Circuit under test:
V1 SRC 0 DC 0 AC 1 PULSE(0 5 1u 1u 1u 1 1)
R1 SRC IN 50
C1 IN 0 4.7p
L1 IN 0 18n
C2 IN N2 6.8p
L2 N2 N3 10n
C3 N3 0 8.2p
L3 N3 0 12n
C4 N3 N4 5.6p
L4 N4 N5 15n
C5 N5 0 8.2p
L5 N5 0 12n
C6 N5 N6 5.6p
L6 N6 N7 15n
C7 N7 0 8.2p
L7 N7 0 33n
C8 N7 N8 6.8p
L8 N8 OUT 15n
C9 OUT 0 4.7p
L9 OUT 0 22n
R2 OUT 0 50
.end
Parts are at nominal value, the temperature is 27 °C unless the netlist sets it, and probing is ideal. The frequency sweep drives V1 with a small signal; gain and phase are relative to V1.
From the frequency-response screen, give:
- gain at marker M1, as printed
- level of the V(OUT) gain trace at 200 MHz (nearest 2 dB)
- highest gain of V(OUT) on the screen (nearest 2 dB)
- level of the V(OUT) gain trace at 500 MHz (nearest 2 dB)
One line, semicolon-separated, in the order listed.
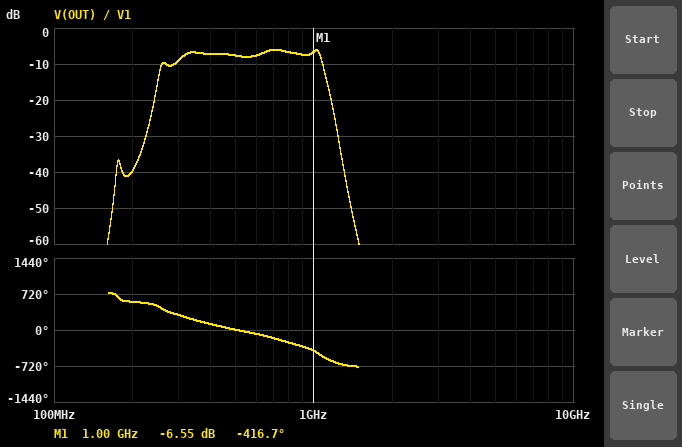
-6.55 dB; -40 dB; -6 dB; -8 dB
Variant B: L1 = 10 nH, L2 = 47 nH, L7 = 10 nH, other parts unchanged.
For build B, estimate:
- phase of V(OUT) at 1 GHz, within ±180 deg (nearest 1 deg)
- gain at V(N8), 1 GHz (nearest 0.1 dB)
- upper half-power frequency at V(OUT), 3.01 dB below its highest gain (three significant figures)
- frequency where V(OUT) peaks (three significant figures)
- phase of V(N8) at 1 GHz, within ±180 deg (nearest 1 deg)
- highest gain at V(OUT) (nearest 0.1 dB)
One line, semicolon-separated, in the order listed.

-129 deg; -12.8 dB; 746 MHz; 401 MHz; -9 deg; -10.5 dB
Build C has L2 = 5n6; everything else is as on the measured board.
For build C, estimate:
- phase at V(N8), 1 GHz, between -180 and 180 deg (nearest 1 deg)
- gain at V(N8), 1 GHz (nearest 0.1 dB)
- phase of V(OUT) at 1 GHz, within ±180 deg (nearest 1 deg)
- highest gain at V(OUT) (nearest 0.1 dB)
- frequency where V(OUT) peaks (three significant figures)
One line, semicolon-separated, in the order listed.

98 deg; -2.2 dB; -23 deg; -6.2 dB; 706 MHz
